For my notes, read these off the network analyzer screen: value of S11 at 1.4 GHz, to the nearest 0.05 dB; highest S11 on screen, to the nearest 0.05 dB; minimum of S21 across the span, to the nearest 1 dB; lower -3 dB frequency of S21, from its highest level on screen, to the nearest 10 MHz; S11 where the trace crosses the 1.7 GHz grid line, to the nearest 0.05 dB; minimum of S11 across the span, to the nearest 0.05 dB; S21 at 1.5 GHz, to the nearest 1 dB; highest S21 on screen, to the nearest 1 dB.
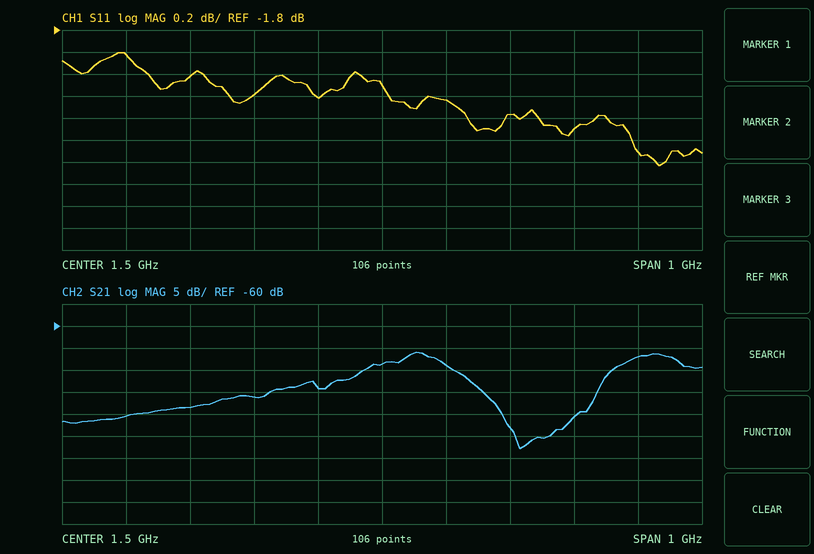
-2.40 dB
-2.00 dB
-88 dB
1.48 GHz
-2.55 dB
-3.05 dB
-69 dB
-66 dB
